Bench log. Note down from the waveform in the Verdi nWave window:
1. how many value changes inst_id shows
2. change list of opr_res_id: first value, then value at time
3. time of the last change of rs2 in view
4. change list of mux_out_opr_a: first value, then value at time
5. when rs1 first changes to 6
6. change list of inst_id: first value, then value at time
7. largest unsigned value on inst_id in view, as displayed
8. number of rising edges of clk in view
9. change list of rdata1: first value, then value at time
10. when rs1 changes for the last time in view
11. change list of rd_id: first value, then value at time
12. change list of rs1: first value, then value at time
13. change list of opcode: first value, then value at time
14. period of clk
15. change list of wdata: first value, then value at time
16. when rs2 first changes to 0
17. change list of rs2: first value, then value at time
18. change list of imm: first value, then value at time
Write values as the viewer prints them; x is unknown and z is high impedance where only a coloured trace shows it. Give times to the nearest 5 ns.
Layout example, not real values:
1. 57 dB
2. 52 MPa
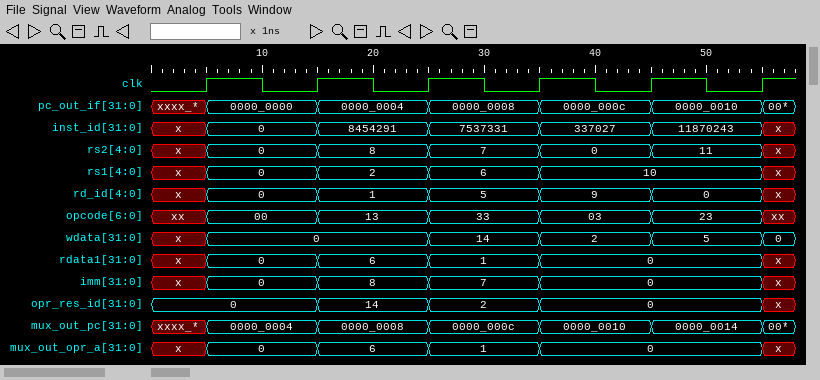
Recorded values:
1. 6
2. 0, 14 at 15 ns, 2 at 25 ns, 0 at 35 ns, x at 55 ns
3. 55 ns
4. x, 0 at 5 ns, 6 at 15 ns, 1 at 25 ns, 0 at 35 ns, x at 55 ns
5. 25 ns
6. x, 0 at 5 ns, 8454291 at 15 ns, 7537331 at 25 ns, 337027 at 35 ns, 11870243 at 45 ns, x at 55 ns
7. 11870243
8. 6
9. x, 0 at 5 ns, 6 at 15 ns, 1 at 25 ns, 0 at 35 ns, x at 55 ns
10. 55 ns
11. x, 0 at 5 ns, 1 at 15 ns, 5 at 25 ns, 9 at 35 ns, 0 at 45 ns, x at 55 ns
12. x, 0 at 5 ns, 2 at 15 ns, 6 at 25 ns, 10 at 35 ns, x at 55 ns
13. xx, 00 at 5 ns, 13 at 15 ns, 33 at 25 ns, 03 at 35 ns, 23 at 45 ns, xx at 55 ns
14. 10 ns
15. x, 0 at 5 ns, 14 at 25 ns, 2 at 35 ns, 5 at 45 ns, 0 at 55 ns
16. 5 ns
17. x, 0 at 5 ns, 8 at 15 ns, 7 at 25 ns, 0 at 35 ns, 11 at 45 ns, x at 55 ns
18. x, 0 at 5 ns, 8 at 15 ns, 7 at 25 ns, 0 at 35 ns, x at 55 ns
